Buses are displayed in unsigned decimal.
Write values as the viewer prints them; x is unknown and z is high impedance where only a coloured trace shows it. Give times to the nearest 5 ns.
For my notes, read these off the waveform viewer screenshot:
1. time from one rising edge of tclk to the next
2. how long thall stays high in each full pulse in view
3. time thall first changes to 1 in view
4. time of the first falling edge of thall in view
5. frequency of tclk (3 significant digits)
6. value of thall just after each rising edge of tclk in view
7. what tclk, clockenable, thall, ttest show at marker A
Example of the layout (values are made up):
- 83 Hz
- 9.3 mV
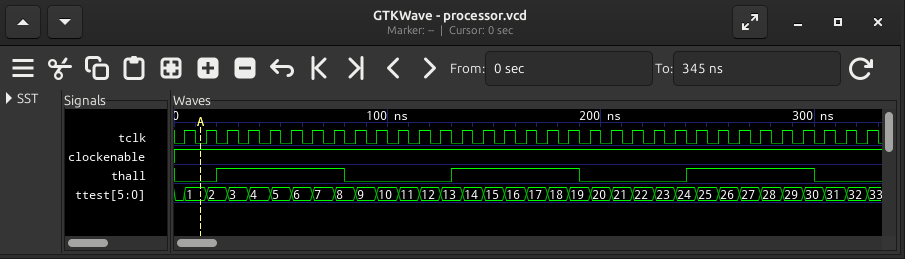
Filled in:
- 10 ns
- 60 ns, 60 ns, 60 ns
- 20 ns
- 80 ns
- 100 MHz
- 0 0 1 1 1 1 1 1 0 0 0 0 0 1 1 1 1 1 1 0 0 0 0 0 1 1 1 1 1 1 0 0 0
- tclk=0, clockenable=1, thall=0, ttest=1
